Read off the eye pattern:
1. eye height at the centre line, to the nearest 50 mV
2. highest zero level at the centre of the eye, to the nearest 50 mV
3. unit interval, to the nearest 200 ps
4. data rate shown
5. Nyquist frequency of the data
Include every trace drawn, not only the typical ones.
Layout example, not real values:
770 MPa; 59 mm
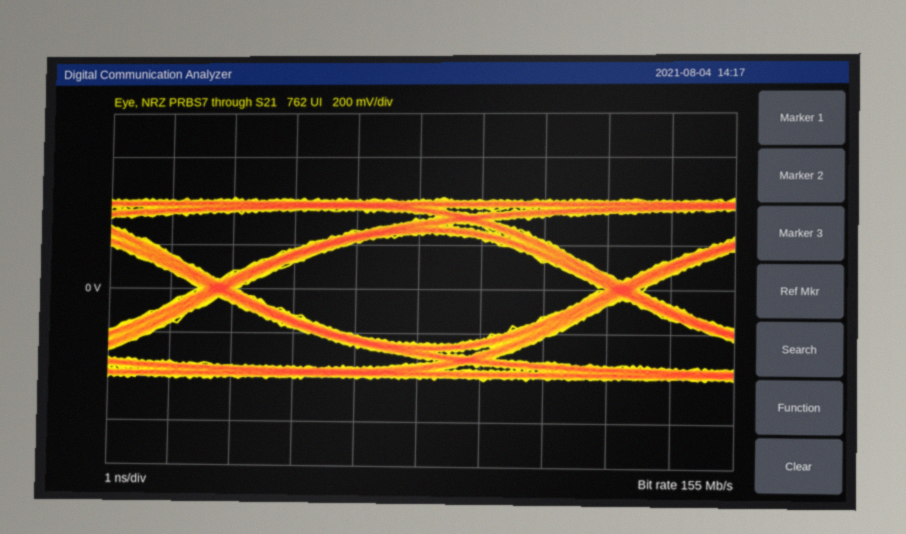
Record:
500 mV; -250 mV; 6.4 ns; 155 Mb/s; 77.5 MHz
